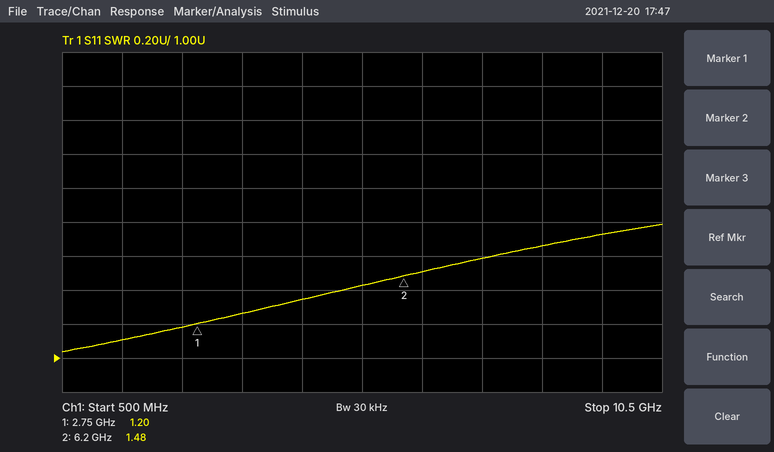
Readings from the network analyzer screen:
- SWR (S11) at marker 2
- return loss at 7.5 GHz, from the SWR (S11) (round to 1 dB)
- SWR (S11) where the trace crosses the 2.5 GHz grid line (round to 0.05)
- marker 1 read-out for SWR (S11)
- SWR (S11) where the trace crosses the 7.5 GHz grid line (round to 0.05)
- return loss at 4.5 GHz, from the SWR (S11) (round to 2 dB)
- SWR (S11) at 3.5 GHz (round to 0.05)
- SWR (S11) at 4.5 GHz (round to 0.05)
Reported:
1.48
13 dB
1.20
1.20
1.60
16 dB
1.25
1.35
